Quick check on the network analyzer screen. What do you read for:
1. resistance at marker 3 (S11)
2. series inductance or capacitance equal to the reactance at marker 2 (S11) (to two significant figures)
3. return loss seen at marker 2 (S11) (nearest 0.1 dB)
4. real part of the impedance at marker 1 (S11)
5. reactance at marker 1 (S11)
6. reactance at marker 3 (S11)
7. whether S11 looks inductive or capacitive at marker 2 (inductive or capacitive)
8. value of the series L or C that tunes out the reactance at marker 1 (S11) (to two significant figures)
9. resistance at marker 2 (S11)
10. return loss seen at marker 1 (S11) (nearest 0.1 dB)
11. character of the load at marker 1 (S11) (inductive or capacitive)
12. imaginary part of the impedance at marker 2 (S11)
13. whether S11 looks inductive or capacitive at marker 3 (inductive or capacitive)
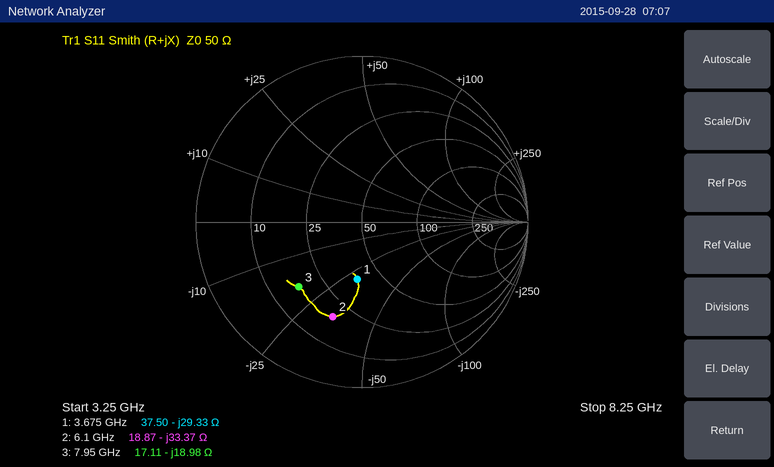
17.11 Ω
780 fF
4.5 dB
37.50 Ω
-29.33 Ω
-18.98 Ω
capacitive
1.3 nH
18.87 Ω
9.2 dB
capacitive
-33.37 Ω
capacitive
